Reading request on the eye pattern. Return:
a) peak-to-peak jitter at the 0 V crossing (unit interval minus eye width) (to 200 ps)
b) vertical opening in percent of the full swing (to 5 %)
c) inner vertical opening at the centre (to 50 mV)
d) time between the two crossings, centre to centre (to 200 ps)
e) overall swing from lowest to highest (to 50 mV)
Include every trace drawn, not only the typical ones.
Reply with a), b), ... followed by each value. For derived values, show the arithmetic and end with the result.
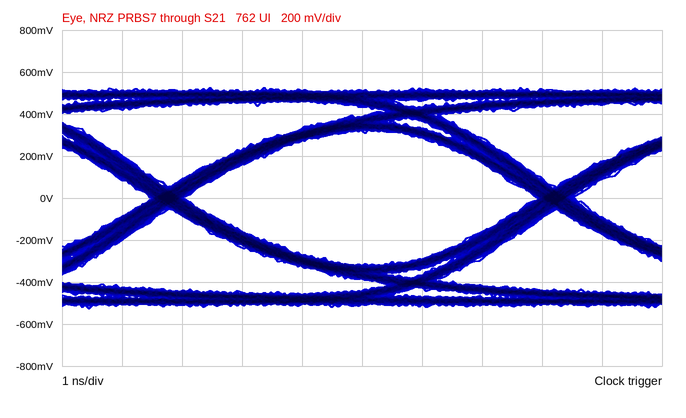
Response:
a) 600 ps
b) 650 mV / 1.05 V ≈ 61.9 %, so 60 % to the nearest 5 %
c) 650 mV
d) 6.4 ns
e) 1.05 V
